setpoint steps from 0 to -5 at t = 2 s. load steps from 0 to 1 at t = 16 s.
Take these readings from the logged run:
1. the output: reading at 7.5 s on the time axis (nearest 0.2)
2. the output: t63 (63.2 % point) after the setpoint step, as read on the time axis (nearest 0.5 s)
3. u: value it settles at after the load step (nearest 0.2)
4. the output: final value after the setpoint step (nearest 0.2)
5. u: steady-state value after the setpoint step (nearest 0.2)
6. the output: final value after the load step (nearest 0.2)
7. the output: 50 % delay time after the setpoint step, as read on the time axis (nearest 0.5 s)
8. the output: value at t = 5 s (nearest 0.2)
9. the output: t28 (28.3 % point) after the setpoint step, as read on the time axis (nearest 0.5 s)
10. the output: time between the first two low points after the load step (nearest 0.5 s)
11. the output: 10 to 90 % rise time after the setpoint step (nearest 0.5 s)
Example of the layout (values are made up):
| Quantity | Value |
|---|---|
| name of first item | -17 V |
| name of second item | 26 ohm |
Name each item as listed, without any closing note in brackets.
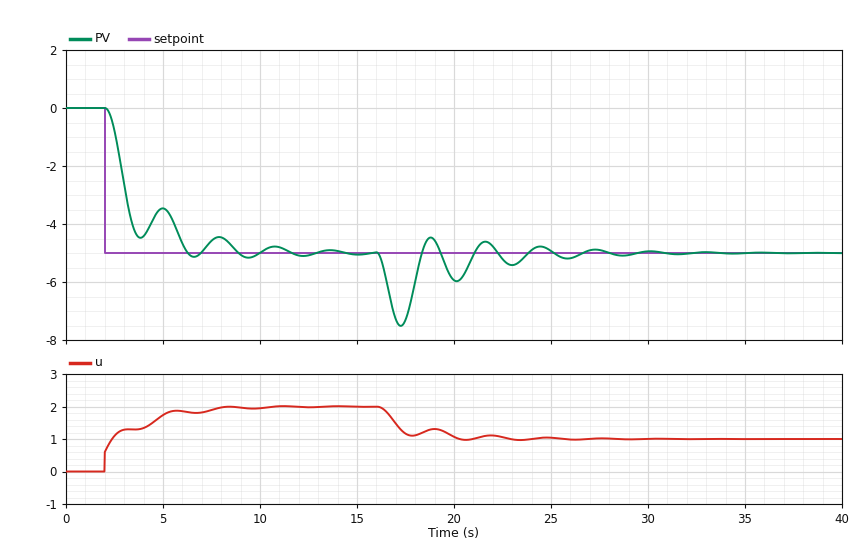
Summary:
| Quantity | Value |
|---|---|
| the output: reading at 7.5 s on the time axis | -4.6 |
| the output: t63 (63.2 % point) after the setpoint step, as read on the time axis | 3.0 s |
| u: value it settles at after the load step | 1.0 |
| the output: final value after the setpoint step | -5.0 |
| u: steady-state value after the setpoint step | 2.0 |
| the output: final value after the load step | -5.0 |
| the output: 50 % delay time after the setpoint step, as read on the time axis | 3.0 s |
| the output: value at t = 5 s | -3.4 |
| the output: t28 (28.3 % point) after the setpoint step, as read on the time axis | 2.5 s |
| the output: time between the first two low points after the load step | 3.0 s |
| the output: 10 to 90 % rise time after the setpoint step | 3.5 s |
